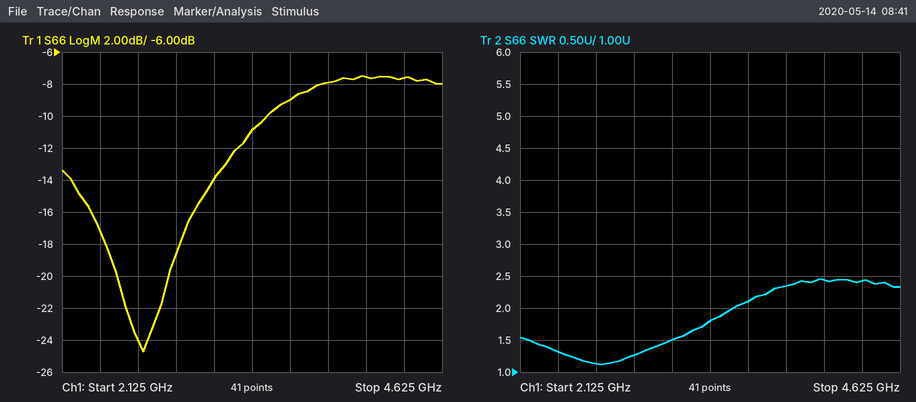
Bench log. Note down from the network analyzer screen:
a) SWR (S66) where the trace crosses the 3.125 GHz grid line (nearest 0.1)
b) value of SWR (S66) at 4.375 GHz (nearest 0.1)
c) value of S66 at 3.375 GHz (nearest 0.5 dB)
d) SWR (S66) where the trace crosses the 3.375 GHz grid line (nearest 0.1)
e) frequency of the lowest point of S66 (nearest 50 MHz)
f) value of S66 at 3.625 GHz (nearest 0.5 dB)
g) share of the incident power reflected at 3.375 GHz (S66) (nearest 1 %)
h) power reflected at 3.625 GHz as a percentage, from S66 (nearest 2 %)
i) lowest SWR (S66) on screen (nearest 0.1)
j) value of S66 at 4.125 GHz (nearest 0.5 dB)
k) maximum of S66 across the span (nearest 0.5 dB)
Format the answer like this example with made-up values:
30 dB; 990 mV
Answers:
1.5; 2.4; -11.0 dB; 1.8; 2.65 GHz; -9.0 dB; 8 %; 12 %; 1.1; -7.5 dB; -7.5 dB
